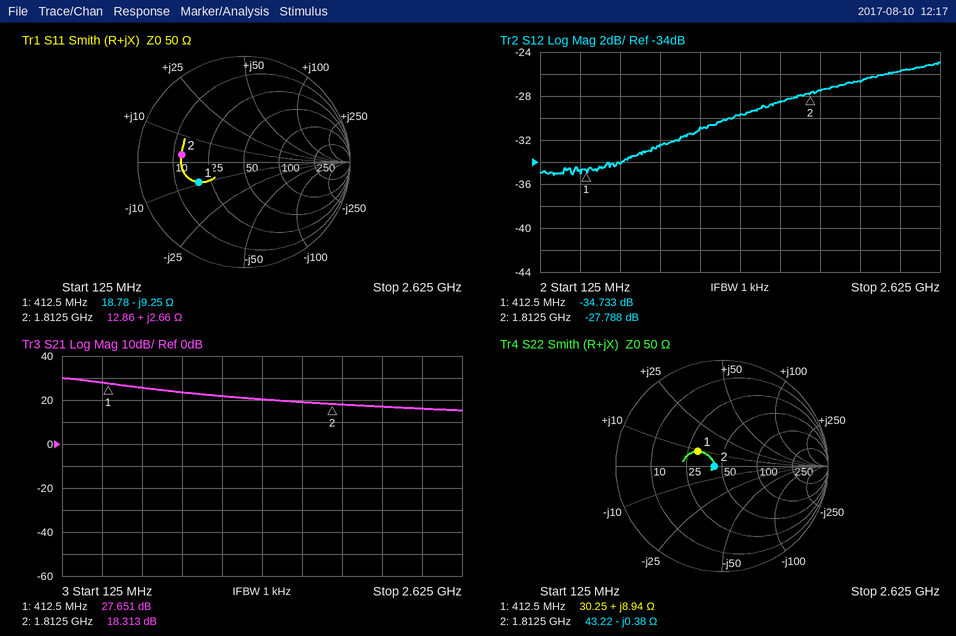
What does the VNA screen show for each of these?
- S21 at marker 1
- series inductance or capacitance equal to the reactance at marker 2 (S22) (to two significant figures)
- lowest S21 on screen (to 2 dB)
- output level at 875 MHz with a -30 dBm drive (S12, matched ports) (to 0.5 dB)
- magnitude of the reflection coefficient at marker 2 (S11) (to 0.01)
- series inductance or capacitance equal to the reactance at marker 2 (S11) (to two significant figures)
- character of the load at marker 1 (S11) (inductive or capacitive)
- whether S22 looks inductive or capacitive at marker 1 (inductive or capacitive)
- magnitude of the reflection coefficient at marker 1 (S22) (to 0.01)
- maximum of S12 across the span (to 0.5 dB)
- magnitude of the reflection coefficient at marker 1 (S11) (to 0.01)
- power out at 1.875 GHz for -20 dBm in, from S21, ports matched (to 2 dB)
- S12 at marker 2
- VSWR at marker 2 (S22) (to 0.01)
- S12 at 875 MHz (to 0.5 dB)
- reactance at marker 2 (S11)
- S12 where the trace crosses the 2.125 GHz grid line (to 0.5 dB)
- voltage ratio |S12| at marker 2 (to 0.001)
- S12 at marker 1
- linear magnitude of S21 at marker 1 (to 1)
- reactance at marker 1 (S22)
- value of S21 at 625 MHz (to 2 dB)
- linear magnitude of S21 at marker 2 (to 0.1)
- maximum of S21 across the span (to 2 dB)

27.651 dB
230 pF
16 dB
-62.5 dBm
0.59
230 pH
capacitive
inductive
0.27
-25.0 dB
0.47
-2 dBm
-27.788 dB
1.16
-32.5 dB
+2.66 Ω
-26.5 dB
0.041
-34.733 dB
24
+8.94 Ω
26 dB
8.2
30 dB
